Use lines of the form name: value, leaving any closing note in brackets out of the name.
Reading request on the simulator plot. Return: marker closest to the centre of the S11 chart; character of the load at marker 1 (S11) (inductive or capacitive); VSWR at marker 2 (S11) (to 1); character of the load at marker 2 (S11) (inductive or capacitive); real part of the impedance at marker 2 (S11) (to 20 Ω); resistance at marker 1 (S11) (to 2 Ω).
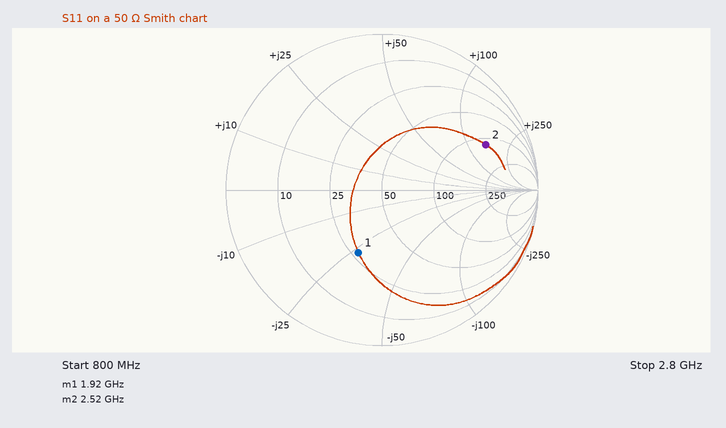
marker closest to the centre of the S11 chart: marker 1
character of the load at marker 1 (S11): capacitive
VSWR at marker 2 (S11): 6
character of the load at marker 2 (S11): inductive
real part of the impedance at marker 2 (S11): 120 Ω
resistance at marker 1 (S11): 28 Ω
